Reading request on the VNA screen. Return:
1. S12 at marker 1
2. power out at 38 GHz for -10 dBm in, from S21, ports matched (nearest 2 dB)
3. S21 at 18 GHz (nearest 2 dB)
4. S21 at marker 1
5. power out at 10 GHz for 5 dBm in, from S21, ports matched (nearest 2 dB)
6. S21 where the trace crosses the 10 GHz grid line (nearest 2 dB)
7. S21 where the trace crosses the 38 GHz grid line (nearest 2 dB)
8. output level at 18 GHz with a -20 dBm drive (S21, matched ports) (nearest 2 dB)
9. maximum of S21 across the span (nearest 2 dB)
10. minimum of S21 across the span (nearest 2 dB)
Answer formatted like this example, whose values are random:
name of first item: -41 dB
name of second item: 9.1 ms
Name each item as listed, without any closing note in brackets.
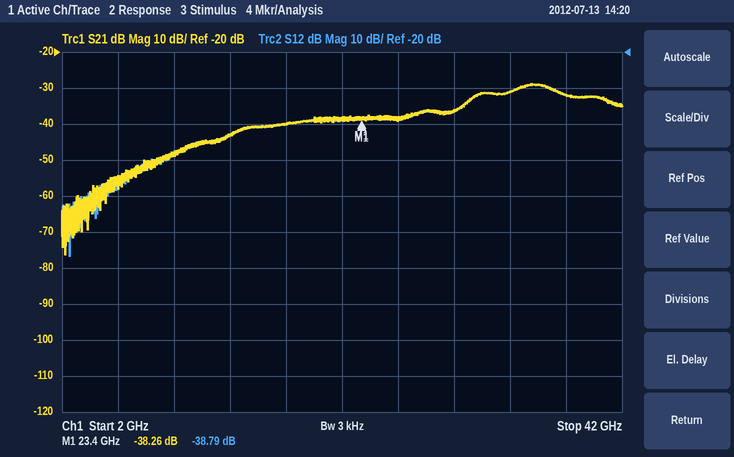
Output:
S12 at marker 1: -38.79 dB
power out at 38 GHz for -10 dBm in, from S21, ports matched: -42 dBm
S21 at 18 GHz: -40 dB
S21 at marker 1: -38.26 dB
power out at 10 GHz for 5 dBm in, from S21, ports matched: -44 dBm
S21 where the trace crosses the 10 GHz grid line: -48 dB
S21 where the trace crosses the 38 GHz grid line: -32 dB
output level at 18 GHz with a -20 dBm drive (S21, matched ports): -60 dBm
maximum of S21 across the span: -28 dB
minimum of S21 across the span: -76 dB
